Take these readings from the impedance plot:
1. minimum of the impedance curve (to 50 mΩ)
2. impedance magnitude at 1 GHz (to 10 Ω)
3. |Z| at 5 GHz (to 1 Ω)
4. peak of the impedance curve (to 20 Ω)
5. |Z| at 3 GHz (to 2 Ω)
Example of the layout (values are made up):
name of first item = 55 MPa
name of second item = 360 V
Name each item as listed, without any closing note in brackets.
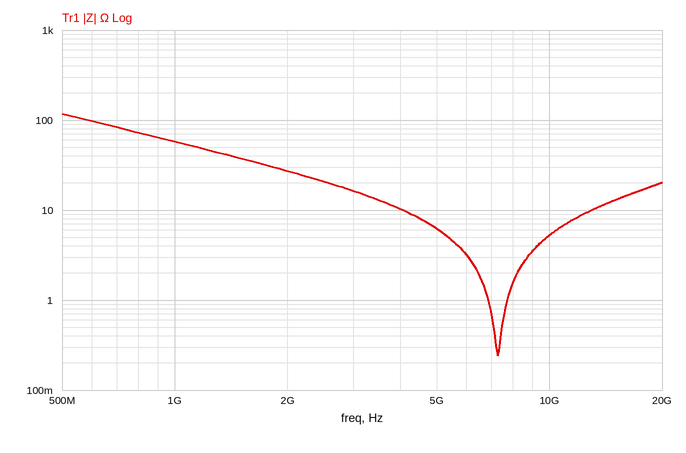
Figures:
minimum of the impedance curve = 250 mΩ
impedance magnitude at 1 GHz = 60 Ω
|Z| at 5 GHz = 6 Ω
peak of the impedance curve = 120 Ω
|Z| at 3 GHz = 16 Ω
